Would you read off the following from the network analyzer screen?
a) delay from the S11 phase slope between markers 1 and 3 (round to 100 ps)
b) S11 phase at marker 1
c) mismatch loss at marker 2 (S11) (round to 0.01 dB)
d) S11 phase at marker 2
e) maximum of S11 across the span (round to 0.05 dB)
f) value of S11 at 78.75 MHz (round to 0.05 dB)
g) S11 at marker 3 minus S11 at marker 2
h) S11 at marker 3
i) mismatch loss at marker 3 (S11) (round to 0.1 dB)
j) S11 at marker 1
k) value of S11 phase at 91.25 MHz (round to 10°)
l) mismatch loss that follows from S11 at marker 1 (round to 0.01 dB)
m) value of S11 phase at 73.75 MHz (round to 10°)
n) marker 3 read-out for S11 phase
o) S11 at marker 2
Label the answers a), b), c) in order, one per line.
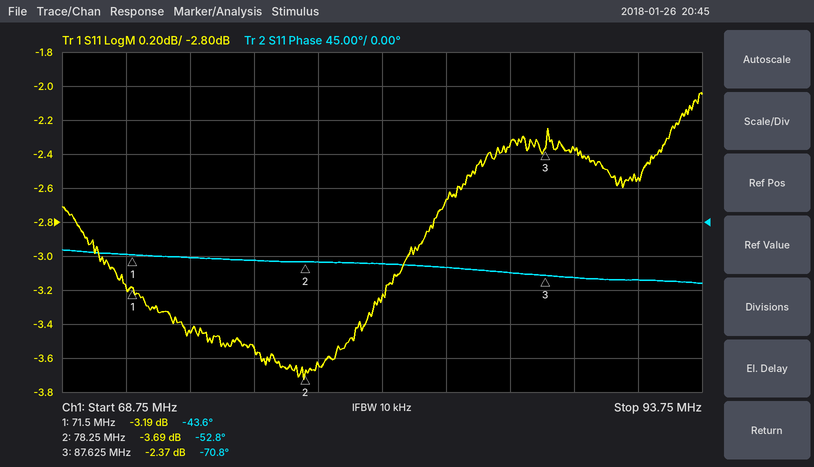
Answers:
a) 4.7 ns
b) -43.6°
c) 2.42 dB
d) -52.8°
e) -2.05 dB
f) -3.65 dB
g) 1.32 dB
h) -2.37 dB
i) 3.8 dB
j) -3.19 dB
k) -80°
l) 2.84 dB
m) -50°
n) -70.8°
o) -3.69 dB
